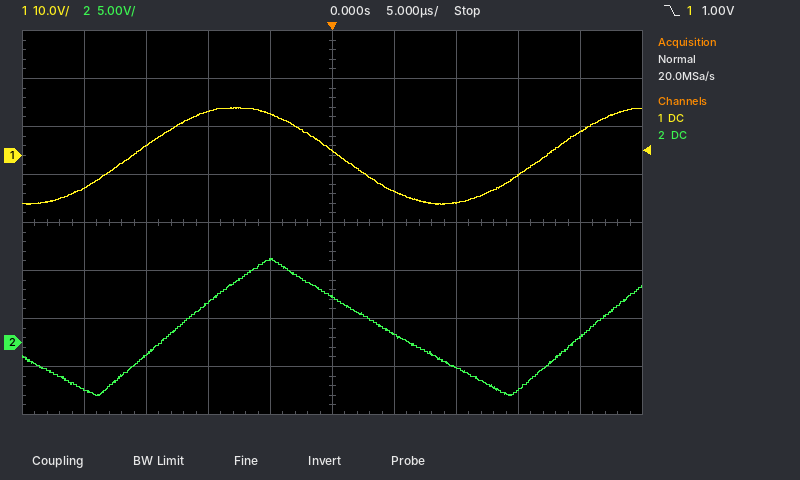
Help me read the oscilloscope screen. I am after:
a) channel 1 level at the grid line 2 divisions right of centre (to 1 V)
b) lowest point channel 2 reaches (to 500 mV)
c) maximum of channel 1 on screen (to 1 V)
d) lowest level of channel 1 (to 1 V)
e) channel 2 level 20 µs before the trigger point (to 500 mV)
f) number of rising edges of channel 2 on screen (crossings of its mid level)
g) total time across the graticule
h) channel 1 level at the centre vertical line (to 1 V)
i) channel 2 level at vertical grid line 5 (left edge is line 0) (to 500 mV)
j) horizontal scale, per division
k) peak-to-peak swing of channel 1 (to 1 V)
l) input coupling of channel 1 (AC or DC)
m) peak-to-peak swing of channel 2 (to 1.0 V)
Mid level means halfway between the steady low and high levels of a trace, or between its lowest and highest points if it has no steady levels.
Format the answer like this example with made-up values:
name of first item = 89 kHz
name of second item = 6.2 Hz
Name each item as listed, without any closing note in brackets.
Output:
channel 1 level at the grid line 2 divisions right of centre = -10 V
lowest point channel 2 reaches = -5.5 V
maximum of channel 1 on screen = 10 V
lowest level of channel 1 = -10 V
channel 2 level 20 µs before the trigger point = -5.0 V
number of rising edges of channel 2 on screen = 2
total time across the graticule = 50 µs
channel 1 level at the centre vertical line = 1 V
channel 2 level at vertical grid line 5 (left edge is line 0) = 4.5 V
horizontal scale, per division = 5 µs
peak-to-peak swing of channel 1 = 20 V
input coupling of channel 1 = DC
peak-to-peak swing of channel 2 = 14.0 V
